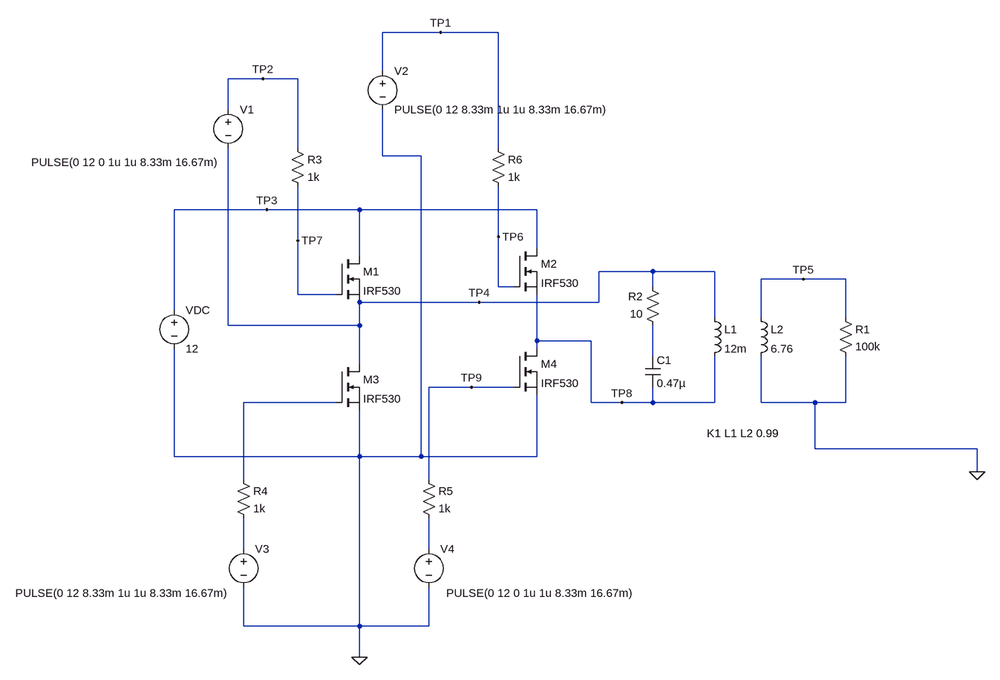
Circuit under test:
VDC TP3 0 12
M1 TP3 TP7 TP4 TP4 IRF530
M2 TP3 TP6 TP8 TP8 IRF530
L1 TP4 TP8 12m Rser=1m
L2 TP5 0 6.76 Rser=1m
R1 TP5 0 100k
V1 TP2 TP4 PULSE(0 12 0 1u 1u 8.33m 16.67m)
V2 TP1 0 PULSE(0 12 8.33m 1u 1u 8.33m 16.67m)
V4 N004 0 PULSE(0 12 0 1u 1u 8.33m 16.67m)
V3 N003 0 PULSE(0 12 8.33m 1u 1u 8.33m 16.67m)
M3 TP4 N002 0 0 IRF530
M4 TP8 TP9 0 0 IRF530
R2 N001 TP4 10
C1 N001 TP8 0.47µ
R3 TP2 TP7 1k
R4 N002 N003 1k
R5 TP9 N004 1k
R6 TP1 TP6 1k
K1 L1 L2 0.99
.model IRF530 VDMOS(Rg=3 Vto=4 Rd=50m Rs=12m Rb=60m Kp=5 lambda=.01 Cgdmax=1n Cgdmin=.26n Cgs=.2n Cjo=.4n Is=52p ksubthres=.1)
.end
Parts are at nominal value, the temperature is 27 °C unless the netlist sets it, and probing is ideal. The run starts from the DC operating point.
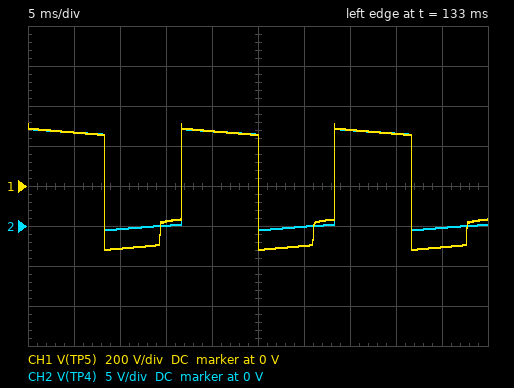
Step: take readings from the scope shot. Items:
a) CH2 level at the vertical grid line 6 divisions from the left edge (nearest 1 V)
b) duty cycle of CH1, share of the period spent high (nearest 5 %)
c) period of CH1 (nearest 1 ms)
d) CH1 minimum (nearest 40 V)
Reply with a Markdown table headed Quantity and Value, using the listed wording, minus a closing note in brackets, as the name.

| Quantity | Value |
|---|---|
| CH2 level at the vertical grid line 6 divisions from the left edge | 0 V |
| duty cycle of CH1, share of the period spent high | 50 % |
| period of CH1 | 17 ms |
| CH1 minimum | -320 V |
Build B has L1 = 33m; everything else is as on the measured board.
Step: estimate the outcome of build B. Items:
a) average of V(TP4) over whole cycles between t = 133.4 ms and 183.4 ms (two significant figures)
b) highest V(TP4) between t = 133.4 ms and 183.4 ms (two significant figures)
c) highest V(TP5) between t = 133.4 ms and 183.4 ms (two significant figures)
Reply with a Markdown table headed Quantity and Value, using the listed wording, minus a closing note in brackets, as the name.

| Quantity | Value |
|---|---|
| average of V(TP4) over whole cycles between t = 133.4 ms and 183.4 ms | 5.9 V |
| highest V(TP4) between t = 133.4 ms and 183.4 ms | 12 V |
| highest V(TP5) between t = 133.4 ms and 183.4 ms | 170 V |
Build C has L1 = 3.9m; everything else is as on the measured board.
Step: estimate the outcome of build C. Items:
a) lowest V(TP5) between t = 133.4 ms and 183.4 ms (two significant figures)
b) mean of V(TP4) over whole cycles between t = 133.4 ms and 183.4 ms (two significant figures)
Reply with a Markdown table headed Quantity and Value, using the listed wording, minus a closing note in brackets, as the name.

| Quantity | Value |
|---|---|
| lowest V(TP5) between t = 133.4 ms and 183.4 ms | -610 V |
| mean of V(TP4) over whole cycles between t = 133.4 ms and 183.4 ms | 5.6 V |
